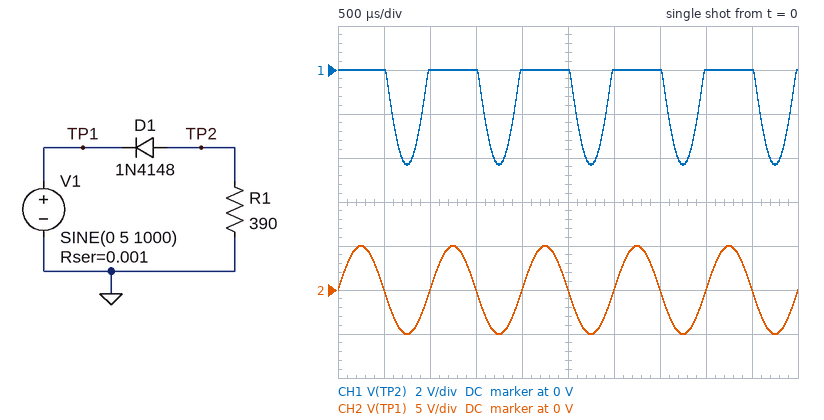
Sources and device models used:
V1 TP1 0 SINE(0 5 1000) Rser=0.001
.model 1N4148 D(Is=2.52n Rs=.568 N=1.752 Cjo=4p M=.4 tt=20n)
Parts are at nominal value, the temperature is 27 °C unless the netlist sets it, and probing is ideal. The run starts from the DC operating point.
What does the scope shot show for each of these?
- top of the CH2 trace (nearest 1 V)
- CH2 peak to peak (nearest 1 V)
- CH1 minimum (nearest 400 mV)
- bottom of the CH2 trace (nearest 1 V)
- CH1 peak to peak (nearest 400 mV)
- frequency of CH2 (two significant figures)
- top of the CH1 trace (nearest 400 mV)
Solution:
5 V
10 V
-4.4 V
-5 V
4.4 V
1.0 kHz
0 V
